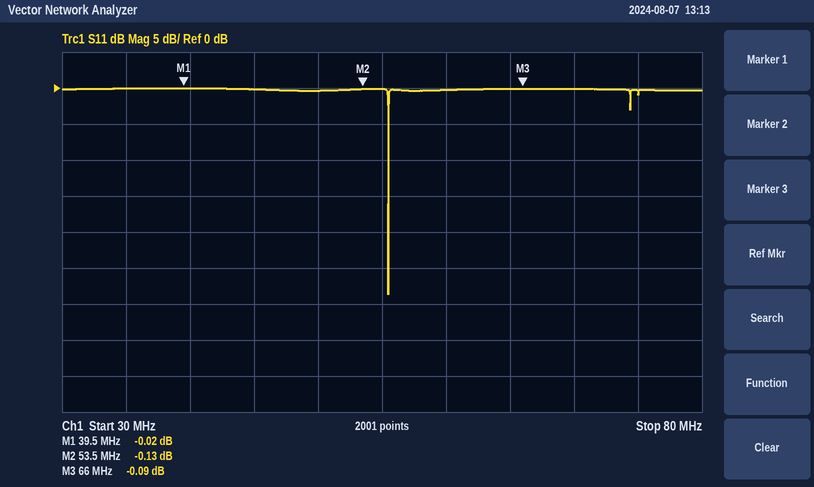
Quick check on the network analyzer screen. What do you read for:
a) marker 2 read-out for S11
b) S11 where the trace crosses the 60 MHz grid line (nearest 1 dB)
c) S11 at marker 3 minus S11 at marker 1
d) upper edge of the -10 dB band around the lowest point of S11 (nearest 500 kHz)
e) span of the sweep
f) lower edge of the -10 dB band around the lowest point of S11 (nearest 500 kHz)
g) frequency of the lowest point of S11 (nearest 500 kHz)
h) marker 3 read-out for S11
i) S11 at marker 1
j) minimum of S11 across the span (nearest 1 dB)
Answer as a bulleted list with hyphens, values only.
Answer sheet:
- -0.13 dB
- 0 dB
- -0.07 dB
- 55.5 MHz
- 50 MHz
- 55.5 MHz
- 55.5 MHz
- -0.09 dB
- -0.02 dB
- -29 dB
